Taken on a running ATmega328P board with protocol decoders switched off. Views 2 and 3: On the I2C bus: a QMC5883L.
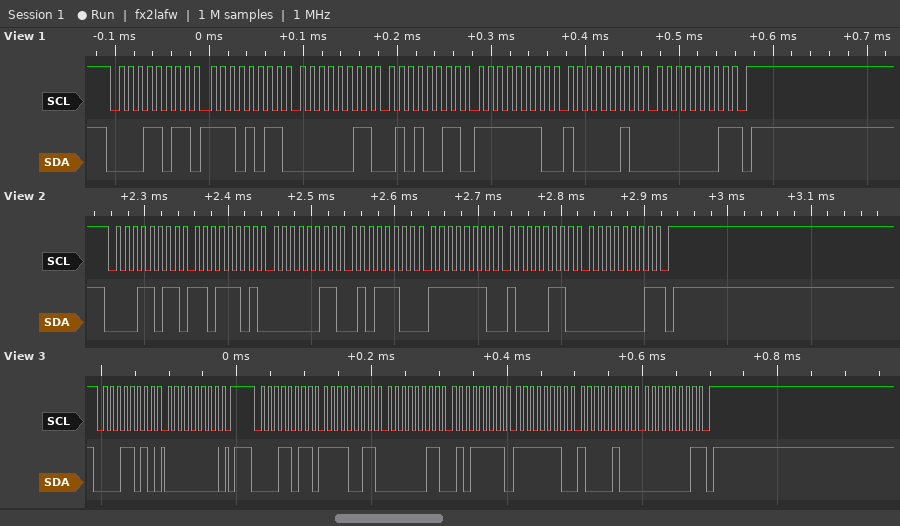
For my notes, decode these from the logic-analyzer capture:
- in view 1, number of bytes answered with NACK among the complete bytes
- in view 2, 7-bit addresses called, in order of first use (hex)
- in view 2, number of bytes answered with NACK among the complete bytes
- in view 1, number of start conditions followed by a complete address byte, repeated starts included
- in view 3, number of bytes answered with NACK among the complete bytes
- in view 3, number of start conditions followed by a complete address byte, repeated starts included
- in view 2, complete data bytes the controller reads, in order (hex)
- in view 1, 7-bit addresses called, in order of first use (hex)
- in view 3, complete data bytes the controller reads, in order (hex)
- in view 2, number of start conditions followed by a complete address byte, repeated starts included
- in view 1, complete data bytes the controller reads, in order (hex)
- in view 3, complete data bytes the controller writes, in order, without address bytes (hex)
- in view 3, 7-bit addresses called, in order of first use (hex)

1
0x0D
1
1
1
2
DD 03 5C FE 86 01
0x0D
F3 03 5F FE 84 01
1
EB 03 53 FE 82 01
00
0x0D
